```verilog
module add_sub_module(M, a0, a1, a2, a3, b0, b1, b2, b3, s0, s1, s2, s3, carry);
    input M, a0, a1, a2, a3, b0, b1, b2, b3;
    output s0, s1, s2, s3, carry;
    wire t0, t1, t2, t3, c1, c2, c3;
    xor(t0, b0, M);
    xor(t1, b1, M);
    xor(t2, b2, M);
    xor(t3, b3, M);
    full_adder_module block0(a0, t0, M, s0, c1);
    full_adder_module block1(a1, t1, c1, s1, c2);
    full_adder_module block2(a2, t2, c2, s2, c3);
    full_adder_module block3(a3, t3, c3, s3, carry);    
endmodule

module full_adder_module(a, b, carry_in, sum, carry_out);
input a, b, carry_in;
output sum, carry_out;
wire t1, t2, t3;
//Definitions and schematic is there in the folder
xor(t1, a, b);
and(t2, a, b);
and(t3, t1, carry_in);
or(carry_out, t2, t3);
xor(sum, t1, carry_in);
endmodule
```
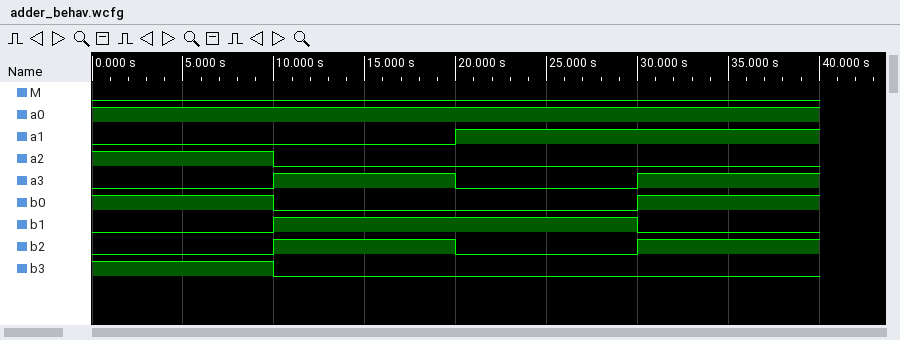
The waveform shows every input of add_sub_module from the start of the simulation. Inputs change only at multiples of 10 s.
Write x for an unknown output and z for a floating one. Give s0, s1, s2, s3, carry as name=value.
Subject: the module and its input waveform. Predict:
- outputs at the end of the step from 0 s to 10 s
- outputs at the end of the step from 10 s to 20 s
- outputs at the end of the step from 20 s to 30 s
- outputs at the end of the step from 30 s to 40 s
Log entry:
s0=0, s1=1, s2=1, s3=1, carry=0
s0=1, s1=1, s2=1, s3=1, carry=0
s0=1, s1=0, s2=1, s3=0, carry=0
s0=0, s1=0, s2=0, s3=0, carry=1
